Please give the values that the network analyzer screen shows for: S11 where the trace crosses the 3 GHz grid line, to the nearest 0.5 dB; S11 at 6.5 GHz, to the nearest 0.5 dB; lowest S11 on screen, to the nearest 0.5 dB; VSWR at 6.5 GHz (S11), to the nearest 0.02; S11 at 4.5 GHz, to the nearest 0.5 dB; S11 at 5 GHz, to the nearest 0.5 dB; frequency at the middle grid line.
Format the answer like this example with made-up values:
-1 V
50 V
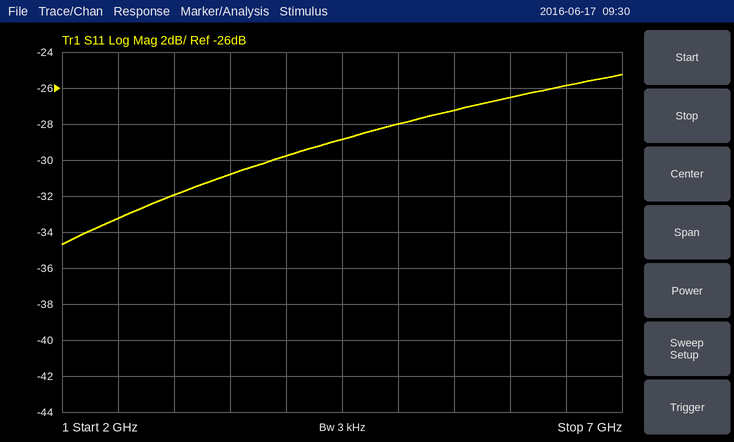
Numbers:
-32.0 dB
-26.0 dB
-34.5 dB
1.10
-29.0 dB
-28.0 dB
4.5 GHz
